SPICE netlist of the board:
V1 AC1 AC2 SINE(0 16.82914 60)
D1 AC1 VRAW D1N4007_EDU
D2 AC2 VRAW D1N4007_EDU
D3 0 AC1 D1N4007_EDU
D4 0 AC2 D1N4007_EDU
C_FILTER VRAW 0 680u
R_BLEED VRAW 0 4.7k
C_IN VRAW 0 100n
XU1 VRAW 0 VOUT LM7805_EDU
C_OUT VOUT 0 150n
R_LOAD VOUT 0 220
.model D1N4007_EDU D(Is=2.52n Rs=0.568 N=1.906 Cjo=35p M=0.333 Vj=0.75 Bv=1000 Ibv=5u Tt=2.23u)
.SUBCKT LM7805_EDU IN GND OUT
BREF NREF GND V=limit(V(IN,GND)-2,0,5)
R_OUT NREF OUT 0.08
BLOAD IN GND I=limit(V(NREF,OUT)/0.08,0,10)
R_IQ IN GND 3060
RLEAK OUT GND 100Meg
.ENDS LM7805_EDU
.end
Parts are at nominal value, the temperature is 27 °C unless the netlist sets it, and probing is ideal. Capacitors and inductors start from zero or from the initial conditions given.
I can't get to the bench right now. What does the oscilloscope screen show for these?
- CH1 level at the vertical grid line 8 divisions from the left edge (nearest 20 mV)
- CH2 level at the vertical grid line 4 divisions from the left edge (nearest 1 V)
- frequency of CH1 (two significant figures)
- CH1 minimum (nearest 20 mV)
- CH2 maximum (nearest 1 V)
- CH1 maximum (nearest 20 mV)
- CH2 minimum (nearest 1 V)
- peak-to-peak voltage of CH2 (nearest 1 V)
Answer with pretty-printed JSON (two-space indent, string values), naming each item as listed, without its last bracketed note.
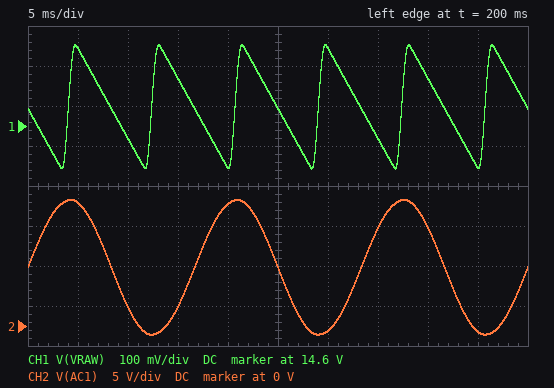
{
  "CH1 level at the vertical grid line 8 divisions from the left edge": "14.72 V",
  "CH2 level at the vertical grid line 4 divisions from the left edge": "15 V",
  "frequency of CH1": "120 Hz",
  "CH1 minimum": "14.50 V",
  "CH2 maximum": "16 V",
  "CH1 maximum": "14.80 V",
  "CH2 minimum": "-1 V",
  "peak-to-peak voltage of CH2": "17 V"
}
